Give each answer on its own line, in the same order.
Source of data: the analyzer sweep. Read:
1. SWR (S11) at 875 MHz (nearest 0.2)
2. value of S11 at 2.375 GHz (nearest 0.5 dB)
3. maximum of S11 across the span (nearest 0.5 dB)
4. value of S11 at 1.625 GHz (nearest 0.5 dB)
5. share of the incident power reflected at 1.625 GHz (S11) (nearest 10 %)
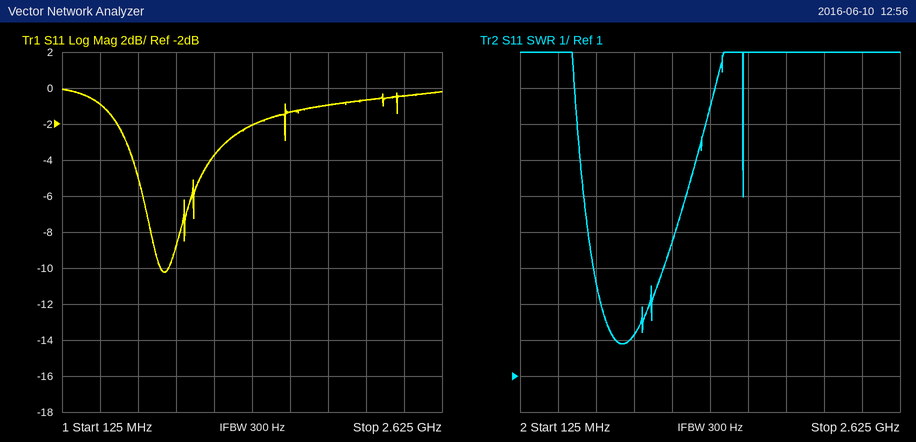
2.2
-0.5 dB
0.0 dB
-1.5 dB
70 %
